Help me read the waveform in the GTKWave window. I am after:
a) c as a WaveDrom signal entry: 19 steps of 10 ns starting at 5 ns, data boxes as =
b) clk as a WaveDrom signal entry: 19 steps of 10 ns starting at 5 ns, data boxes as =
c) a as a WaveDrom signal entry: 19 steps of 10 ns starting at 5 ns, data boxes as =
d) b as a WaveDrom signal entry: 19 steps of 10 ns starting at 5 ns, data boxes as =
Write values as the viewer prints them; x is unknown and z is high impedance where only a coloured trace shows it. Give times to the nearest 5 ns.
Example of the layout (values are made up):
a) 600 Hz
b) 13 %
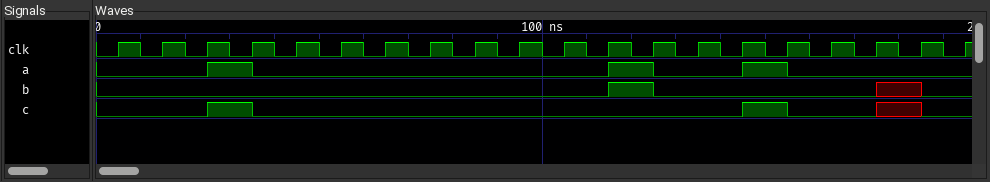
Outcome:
a) {name: 'c', wave: '0.10..........10.x0'}
b) {name: 'clk', wave: 'p..................'}
c) {name: 'a', wave: '0.10.......10.10...'}
d) {name: 'b', wave: '0..........10....x0'}
